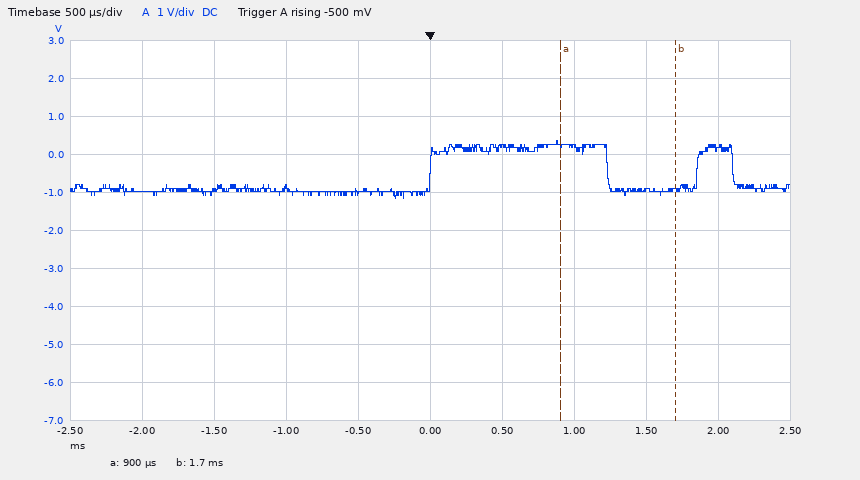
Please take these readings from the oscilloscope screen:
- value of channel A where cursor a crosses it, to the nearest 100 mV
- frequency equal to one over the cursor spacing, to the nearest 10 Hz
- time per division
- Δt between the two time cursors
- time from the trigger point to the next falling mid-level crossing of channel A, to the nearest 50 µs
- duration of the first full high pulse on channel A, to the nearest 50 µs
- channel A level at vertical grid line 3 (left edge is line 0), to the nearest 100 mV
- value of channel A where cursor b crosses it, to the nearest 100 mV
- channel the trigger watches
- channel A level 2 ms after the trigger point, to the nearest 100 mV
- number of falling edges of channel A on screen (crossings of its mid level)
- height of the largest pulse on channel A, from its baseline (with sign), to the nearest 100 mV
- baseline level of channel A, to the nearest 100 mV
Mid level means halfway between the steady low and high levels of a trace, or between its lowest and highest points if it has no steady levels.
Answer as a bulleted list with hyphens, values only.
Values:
- 300 mV
- 1.25 kHz
- 500 µs
- 800 µs
- 1.25 ms
- 1.25 ms
- -900 mV
- -900 mV
- channel A
- 200 mV
- 2
- +1.3 V
- -900 mV
